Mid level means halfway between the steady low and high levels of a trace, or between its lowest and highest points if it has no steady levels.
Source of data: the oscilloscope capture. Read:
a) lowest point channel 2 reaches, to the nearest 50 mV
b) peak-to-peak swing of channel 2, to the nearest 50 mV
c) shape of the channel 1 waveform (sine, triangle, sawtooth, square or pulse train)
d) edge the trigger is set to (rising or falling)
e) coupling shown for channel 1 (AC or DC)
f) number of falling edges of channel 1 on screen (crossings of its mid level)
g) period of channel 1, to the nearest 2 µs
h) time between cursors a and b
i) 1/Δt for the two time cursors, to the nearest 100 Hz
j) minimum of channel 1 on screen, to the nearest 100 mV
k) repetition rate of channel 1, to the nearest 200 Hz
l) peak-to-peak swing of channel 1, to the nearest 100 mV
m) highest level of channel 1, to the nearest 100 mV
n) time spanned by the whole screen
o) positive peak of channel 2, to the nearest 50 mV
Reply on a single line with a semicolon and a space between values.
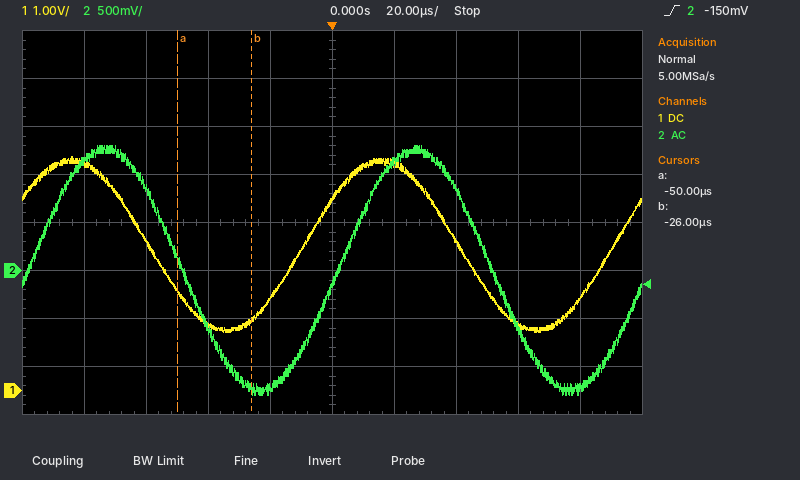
-1.30 V; 2.60 V; sine; rising; DC; 2; 100 µs; 24 µs; 41.7 kHz; 1.2 V; 10.0 kHz; 3.7 V; 4.9 V; 200 µs; 1.30 V
